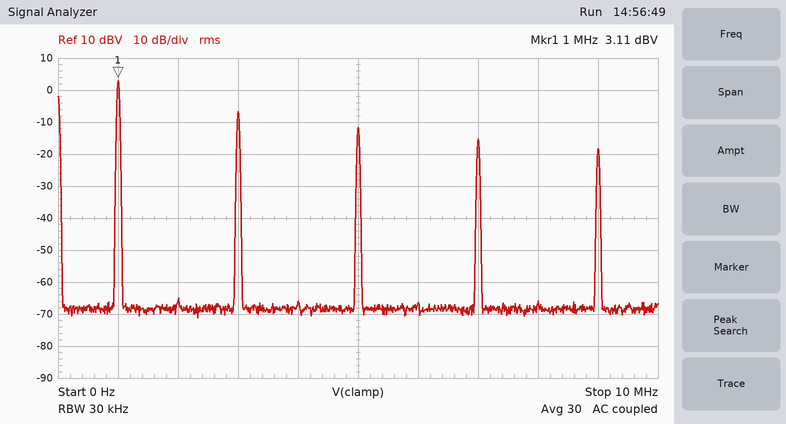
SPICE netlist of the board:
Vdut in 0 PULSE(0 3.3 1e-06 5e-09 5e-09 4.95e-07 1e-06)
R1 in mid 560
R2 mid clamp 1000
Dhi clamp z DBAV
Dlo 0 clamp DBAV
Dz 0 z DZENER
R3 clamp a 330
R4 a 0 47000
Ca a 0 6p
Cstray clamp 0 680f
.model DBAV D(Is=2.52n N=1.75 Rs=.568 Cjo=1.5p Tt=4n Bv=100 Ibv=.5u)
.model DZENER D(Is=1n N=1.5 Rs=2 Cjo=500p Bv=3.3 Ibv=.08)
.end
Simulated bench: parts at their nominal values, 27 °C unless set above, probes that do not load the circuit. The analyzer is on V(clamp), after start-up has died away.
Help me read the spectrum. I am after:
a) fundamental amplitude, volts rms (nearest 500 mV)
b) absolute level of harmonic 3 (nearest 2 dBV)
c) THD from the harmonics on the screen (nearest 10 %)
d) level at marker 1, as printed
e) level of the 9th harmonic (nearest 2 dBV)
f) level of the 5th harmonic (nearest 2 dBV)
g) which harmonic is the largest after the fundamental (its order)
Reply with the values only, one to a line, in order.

1.5 V
-6 dBV
40 %
3.11 dBV
-18 dBV
-12 dBV
3
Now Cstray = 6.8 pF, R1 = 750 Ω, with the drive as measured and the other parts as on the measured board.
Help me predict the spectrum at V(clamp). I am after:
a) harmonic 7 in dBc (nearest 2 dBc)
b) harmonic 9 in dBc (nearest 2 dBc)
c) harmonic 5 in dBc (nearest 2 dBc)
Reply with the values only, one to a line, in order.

-20 dBc
-24 dBc
-16 dBc
